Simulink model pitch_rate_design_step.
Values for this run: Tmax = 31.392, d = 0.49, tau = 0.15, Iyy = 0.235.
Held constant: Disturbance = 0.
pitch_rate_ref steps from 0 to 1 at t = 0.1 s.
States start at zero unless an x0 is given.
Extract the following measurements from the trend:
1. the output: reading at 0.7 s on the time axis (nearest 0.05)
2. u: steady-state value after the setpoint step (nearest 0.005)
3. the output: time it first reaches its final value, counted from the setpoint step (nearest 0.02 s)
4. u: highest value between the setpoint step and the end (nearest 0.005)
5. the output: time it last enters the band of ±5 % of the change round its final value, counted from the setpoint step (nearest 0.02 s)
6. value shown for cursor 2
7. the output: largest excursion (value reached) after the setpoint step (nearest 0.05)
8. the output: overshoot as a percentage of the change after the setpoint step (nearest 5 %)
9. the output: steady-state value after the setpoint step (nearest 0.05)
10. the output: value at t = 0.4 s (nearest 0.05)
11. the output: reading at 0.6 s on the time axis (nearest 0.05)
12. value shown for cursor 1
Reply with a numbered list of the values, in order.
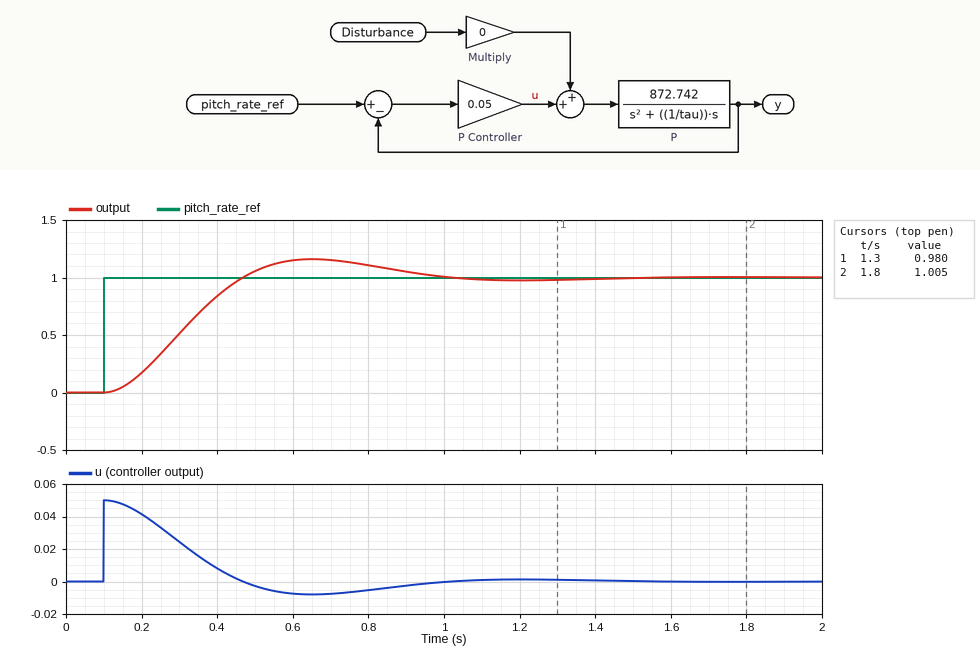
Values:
1. 1.15
2. 0.000
3. 0.36 s
4. 0.050
5. 0.80 s
6. 1.005
7. 1.15
8. 15 %
9. 1.00
10. 0.85
11. 1.15
12. 0.980
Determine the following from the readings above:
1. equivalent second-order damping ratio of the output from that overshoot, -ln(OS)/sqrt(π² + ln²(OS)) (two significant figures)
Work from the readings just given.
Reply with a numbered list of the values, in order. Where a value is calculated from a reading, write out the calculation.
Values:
1. ln(0.15) = -1.897; 1.897 / sqrt(9.870 + 3.599) = 0.52
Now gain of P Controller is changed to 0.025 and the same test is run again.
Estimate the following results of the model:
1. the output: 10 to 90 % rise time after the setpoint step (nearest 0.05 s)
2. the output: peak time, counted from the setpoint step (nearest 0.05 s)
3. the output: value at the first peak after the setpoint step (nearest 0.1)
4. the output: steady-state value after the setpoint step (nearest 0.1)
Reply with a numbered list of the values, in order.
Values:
1. 0.45 s
2. 0.95 s
3. 1.0
4. 1.0
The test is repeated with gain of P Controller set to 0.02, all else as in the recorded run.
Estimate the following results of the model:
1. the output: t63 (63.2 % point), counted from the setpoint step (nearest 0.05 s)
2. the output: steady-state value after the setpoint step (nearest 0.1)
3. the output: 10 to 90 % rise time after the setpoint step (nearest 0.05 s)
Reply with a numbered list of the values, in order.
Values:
1. 0.45 s
2. 1.0
3. 0.60 s
